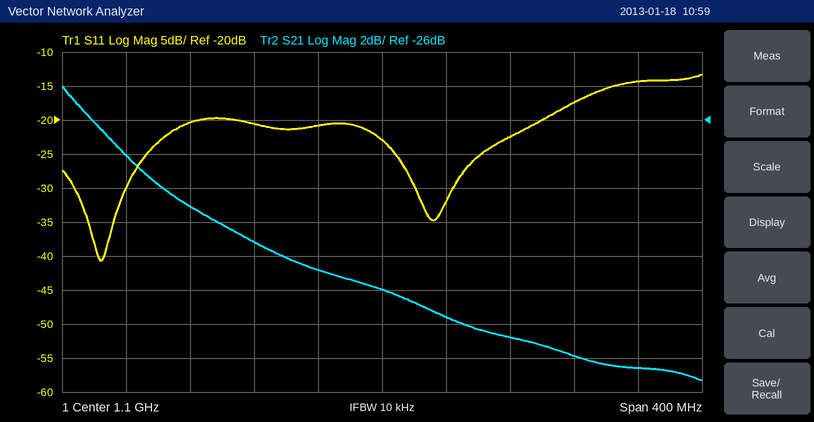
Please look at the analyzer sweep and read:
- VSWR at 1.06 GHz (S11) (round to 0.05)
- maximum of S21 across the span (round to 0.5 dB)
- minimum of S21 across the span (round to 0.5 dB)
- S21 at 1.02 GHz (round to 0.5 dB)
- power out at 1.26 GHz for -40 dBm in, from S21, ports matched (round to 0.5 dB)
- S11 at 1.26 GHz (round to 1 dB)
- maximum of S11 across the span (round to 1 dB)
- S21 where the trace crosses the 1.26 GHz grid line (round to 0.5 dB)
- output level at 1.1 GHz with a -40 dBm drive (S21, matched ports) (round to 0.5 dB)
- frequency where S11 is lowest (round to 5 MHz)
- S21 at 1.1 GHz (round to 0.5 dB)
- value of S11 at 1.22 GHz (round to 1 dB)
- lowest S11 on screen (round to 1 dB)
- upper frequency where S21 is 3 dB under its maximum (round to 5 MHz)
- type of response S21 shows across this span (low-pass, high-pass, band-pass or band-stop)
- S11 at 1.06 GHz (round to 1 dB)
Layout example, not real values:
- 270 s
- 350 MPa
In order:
- 1.20
- -24.0 dB
- -41.5 dB
- -33.0 dB
- -80.5 dBm
- -14 dB
- -13 dB
- -40.5 dB
- -76.0 dBm
- 925 MHz
- -36.0 dB
- -17 dB
- -41 dB
- 930 MHz
- low-pass
- -21 dB
